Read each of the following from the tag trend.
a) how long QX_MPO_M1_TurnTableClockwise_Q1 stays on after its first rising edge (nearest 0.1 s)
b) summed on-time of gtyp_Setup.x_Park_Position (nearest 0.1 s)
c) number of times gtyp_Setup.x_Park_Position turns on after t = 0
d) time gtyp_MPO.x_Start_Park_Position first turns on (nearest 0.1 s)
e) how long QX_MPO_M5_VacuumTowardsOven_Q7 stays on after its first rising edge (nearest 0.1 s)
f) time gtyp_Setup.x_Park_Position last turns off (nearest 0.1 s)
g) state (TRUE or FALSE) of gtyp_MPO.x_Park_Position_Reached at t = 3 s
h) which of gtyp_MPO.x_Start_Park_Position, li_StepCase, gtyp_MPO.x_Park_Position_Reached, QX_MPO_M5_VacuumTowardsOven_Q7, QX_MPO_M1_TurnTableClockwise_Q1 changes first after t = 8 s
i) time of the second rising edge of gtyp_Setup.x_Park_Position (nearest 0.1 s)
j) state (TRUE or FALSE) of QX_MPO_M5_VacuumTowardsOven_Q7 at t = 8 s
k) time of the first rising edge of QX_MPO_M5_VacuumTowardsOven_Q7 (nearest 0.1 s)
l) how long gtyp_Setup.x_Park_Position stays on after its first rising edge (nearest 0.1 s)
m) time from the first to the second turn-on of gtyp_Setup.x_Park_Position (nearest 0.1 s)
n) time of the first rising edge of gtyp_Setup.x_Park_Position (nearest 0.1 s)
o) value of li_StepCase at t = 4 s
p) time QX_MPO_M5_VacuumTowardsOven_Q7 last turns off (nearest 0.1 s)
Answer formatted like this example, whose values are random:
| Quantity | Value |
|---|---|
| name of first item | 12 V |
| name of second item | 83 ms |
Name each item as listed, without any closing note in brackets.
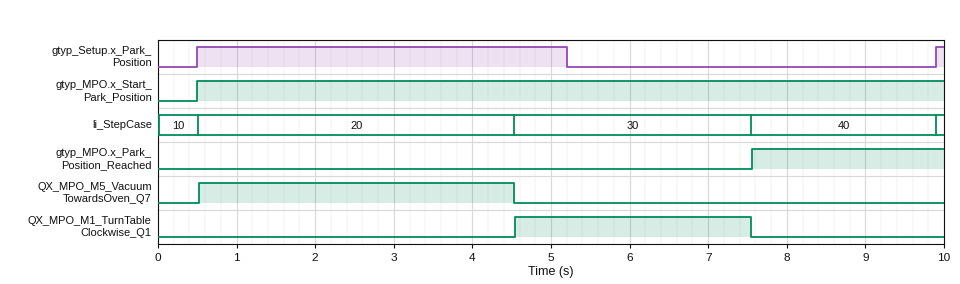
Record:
| Quantity | Value |
|---|---|
| how long QX_MPO_M1_TurnTableClockwise_Q1 stays on after its first rising edge | 3.0 s |
| summed on-time of gtyp_Setup.x_Park_Position | 4.8 s |
| number of times gtyp_Setup.x_Park_Position turns on after t = 0 | 2 |
| time gtyp_MPO.x_Start_Park_Position first turns on | 0.5 s |
| how long QX_MPO_M5_VacuumTowardsOven_Q7 stays on after its first rising edge | 4.0 s |
| time gtyp_Setup.x_Park_Position last turns off | 5.2 s |
| state (TRUE or FALSE) of gtyp_MPO.x_Park_Position_Reached at t = 3 s | FALSE |
| which of gtyp_MPO.x_Start_Park_Position, li_StepCase, gtyp_MPO.x_Park_Position_Reached, QX_MPO_M5_VacuumTowardsOven_Q7, QX_MPO_M1_TurnTableClockwise_Q1 changes first after t = 8 s | li_StepCase |
| time of the second rising edge of gtyp_Setup.x_Park_Position | 9.9 s |
| state (TRUE or FALSE) of QX_MPO_M5_VacuumTowardsOven_Q7 at t = 8 s | FALSE |
| time of the first rising edge of QX_MPO_M5_VacuumTowardsOven_Q7 | 0.5 s |
| how long gtyp_Setup.x_Park_Position stays on after its first rising edge | 4.7 s |
| time from the first to the second turn-on of gtyp_Setup.x_Park_Position | 9.4 s |
| time of the first rising edge of gtyp_Setup.x_Park_Position | 0.5 s |
| value of li_StepCase at t = 4 s | 20 |
| time QX_MPO_M5_VacuumTowardsOven_Q7 last turns off | 4.5 s |
